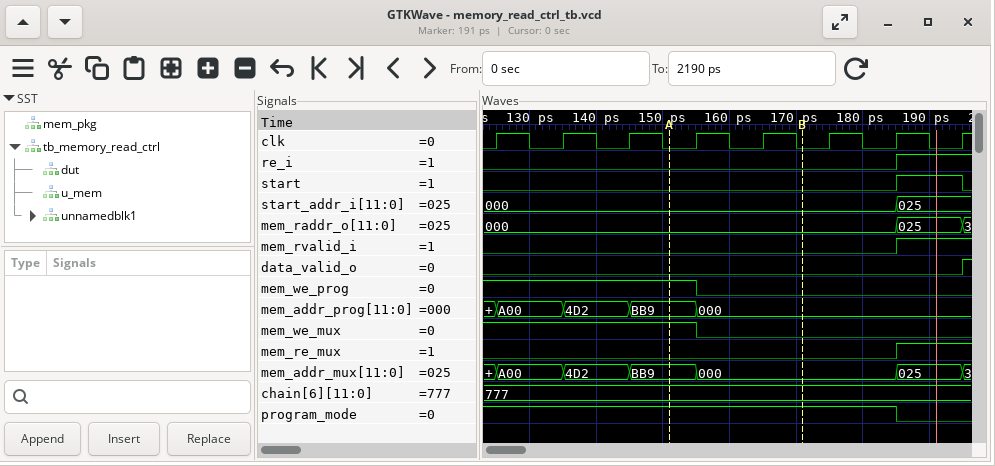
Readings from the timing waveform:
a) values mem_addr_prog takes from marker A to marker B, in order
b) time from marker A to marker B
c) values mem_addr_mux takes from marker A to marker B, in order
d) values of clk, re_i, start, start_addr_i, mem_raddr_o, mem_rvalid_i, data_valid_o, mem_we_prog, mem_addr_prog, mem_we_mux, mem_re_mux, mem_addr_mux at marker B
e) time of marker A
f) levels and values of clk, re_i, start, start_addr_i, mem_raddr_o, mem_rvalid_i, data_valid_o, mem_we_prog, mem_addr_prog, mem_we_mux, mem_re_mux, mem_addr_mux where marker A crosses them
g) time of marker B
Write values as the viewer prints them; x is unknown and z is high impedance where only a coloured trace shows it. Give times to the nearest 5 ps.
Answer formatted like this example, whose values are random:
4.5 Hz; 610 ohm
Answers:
BB9, 000; 20 ps; BB9, 000; clk=0, re_i=0, start=0, start_addr_i=000, mem_raddr_o=000, mem_rvalid_i=0, data_valid_o=0, mem_we_prog=0, mem_addr_prog=000, mem_we_mux=0, mem_re_mux=0, mem_addr_mux=000; 150 ps; clk=0, re_i=0, start=0, start_addr_i=000, mem_raddr_o=000, mem_rvalid_i=0, data_valid_o=0, mem_we_prog=1, mem_addr_prog=BB9, mem_we_mux=1, mem_re_mux=0, mem_addr_mux=BB9; 170 ps
